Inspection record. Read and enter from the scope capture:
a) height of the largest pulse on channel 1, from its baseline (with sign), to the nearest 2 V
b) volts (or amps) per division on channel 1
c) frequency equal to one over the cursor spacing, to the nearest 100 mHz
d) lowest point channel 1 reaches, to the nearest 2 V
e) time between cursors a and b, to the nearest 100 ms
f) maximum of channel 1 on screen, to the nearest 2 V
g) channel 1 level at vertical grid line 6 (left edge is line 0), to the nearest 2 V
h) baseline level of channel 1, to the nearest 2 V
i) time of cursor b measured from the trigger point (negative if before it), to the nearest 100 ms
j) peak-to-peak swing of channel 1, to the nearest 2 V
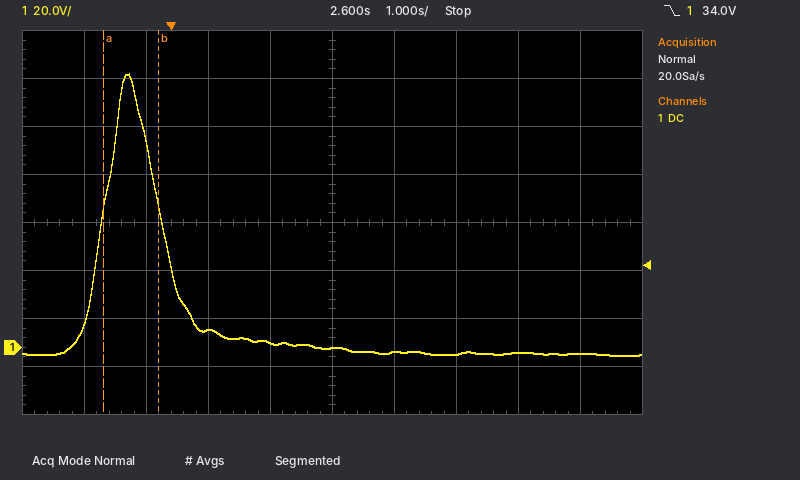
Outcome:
+116 V
20 V
1.1 Hz
-4 V
900 ms
114 V
-2 V
-2 V
-200 ms
118 V
